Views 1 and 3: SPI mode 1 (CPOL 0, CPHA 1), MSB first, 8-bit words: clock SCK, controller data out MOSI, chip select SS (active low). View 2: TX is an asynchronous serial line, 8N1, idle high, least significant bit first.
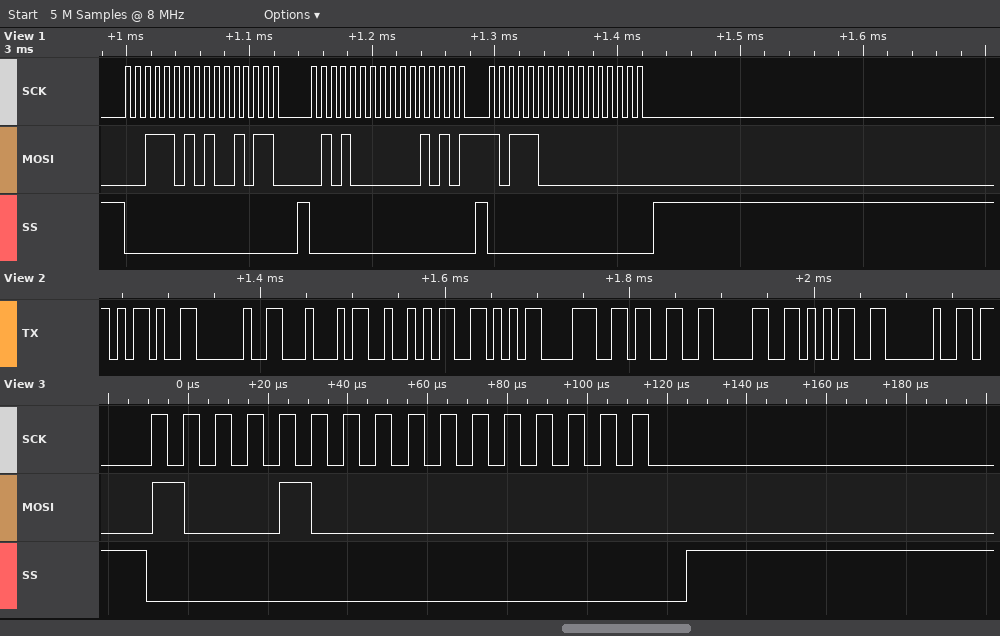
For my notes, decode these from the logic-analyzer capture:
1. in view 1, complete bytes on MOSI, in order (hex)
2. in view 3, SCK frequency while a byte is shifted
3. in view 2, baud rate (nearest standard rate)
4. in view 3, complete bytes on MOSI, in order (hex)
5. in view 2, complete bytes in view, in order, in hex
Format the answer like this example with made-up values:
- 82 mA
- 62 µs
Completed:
- 3A 96 50 15 B8 00
- 125 kHz
- 115200 baud
- 88 00
- 2D 20 44 52 56 38 33 30 35 20
